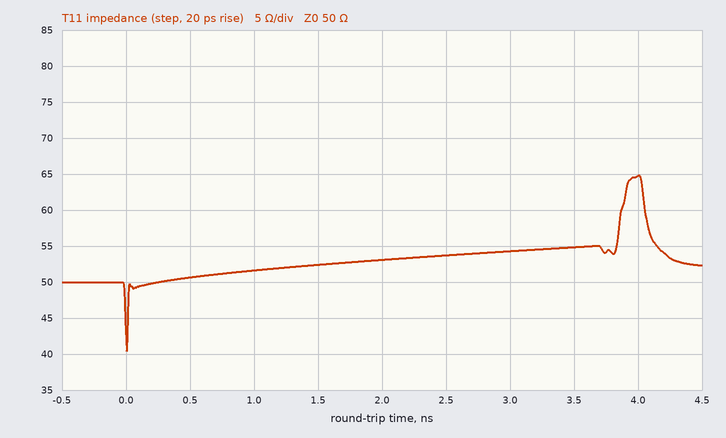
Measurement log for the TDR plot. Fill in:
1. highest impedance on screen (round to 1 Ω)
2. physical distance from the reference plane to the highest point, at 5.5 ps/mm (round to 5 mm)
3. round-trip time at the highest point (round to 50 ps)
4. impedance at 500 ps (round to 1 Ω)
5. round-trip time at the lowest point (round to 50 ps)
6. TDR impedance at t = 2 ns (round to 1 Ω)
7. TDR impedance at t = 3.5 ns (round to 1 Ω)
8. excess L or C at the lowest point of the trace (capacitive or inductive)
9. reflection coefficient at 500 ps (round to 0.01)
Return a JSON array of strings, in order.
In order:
["65 Ω", "365 mm", "4.00 ns", "51 Ω", "0 ps", "53 Ω", "55 Ω", "capacitive", "+0.01"]
